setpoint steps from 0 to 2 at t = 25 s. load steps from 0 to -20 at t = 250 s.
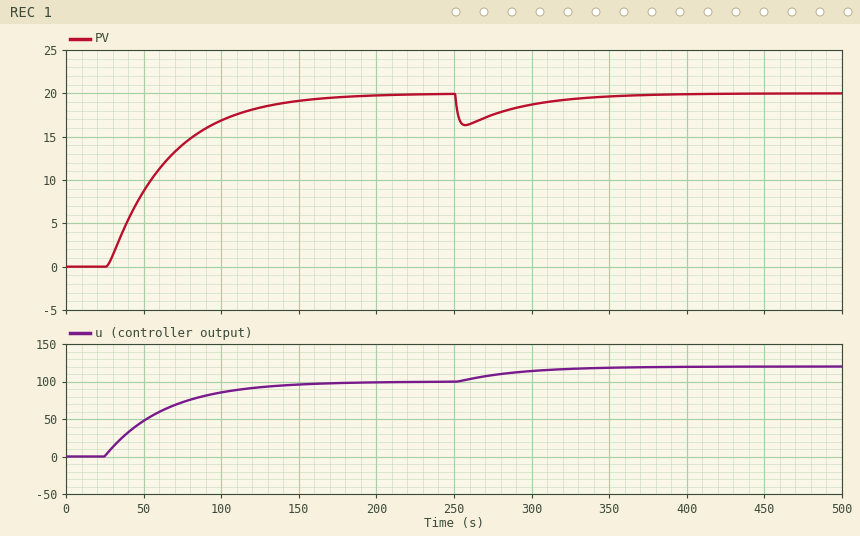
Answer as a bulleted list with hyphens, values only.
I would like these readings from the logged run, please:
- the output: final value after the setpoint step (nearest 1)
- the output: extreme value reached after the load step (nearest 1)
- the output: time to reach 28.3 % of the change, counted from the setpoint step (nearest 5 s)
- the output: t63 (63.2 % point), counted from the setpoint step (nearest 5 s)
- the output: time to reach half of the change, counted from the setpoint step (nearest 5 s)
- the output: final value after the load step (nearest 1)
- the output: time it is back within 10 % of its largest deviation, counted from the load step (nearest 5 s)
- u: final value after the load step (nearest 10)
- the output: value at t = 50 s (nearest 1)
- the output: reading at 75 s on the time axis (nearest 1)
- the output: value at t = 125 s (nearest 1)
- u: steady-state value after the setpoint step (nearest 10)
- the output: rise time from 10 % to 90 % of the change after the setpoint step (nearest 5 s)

- 20
- 16
- 15 s
- 40 s
- 30 s
- 20
- 100 s
- 120
- 9
- 14
- 18
- 100
- 85 s
